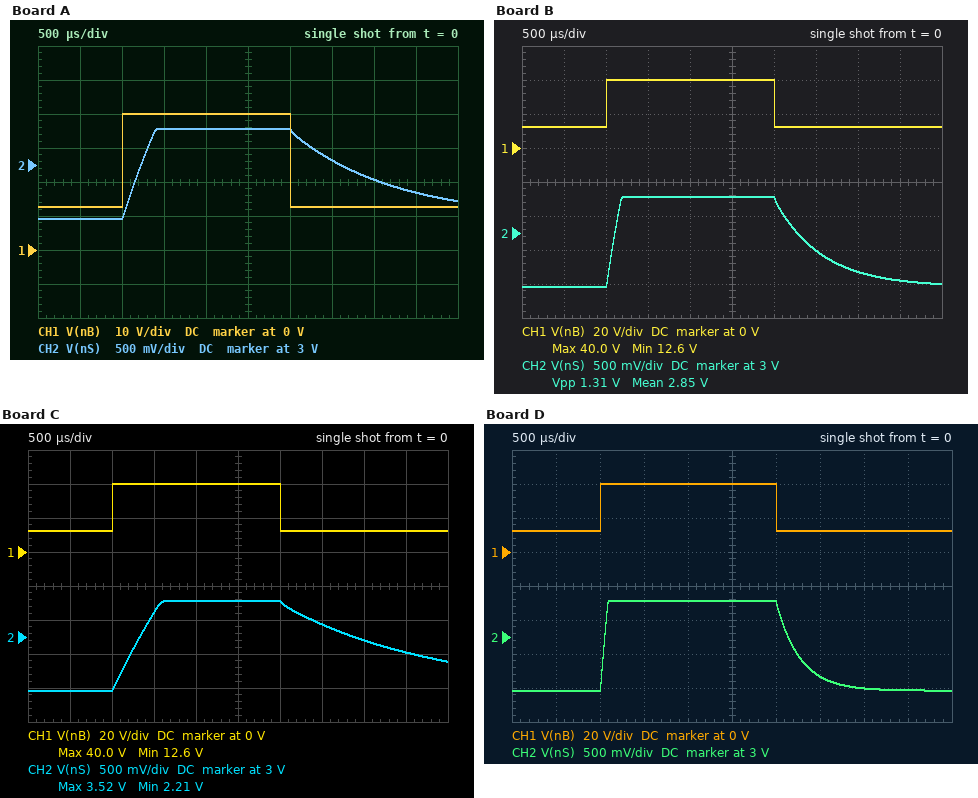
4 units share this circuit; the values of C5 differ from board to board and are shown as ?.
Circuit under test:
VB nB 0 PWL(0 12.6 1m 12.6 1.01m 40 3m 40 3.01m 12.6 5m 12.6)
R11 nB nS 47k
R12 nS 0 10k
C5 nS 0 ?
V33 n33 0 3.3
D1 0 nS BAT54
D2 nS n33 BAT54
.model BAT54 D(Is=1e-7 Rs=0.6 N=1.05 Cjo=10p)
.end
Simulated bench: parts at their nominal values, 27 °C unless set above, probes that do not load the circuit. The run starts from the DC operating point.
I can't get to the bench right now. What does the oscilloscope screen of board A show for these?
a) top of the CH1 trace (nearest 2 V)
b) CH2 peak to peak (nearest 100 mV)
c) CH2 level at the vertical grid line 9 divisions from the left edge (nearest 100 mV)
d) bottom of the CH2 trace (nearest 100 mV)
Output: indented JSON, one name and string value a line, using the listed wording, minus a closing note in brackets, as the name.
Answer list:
{
  "top of the CH1 trace": "40 V",
  "CH2 peak to peak": "1.3 V",
  "CH2 level at the vertical grid line 9 divisions from the left edge": "2.6 V",
  "bottom of the CH2 trace": "2.2 V"
}
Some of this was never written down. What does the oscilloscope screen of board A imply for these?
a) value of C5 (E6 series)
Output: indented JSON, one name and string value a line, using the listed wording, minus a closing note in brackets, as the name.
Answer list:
{
  "value of C5": "150 nF"
}
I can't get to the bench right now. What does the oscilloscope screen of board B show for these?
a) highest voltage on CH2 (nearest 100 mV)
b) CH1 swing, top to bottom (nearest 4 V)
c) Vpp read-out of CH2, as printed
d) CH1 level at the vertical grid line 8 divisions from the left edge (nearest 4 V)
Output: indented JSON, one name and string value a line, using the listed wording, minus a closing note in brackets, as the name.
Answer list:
{
  "highest voltage on CH2": "3.5 V",
  "CH1 swing, top to bottom": "28 V",
  "Vpp read-out of CH2, as printed": "1.31 V",
  "CH1 level at the vertical grid line 8 divisions from the left edge": "12 V"
}
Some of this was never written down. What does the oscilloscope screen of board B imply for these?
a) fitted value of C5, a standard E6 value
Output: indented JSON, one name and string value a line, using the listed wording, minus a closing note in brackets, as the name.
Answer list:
{
  "fitted value of C5, a standard E6 value": "68 nF"
}
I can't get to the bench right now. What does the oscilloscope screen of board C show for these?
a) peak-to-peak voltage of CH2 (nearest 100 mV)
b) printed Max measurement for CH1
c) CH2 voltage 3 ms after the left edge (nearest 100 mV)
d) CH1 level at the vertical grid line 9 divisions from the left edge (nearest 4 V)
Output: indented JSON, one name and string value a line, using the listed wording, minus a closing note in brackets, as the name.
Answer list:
{
  "peak-to-peak voltage of CH2": "1.3 V",
  "printed Max measurement for CH1": "40.0 V",
  "CH2 voltage 3 ms after the left edge": "3.5 V",
  "CH1 level at the vertical grid line 9 divisions from the left edge": "12 V"
}
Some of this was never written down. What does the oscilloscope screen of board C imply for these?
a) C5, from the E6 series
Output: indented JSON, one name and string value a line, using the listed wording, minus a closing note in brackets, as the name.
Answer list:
{
  "C5, from the E6 series": "220 nF"
}
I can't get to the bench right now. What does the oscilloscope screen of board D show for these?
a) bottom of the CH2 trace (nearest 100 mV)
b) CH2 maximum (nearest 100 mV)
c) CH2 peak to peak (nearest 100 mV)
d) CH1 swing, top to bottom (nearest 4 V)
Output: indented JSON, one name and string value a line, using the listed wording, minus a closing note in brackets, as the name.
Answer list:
{
  "bottom of the CH2 trace": "2.2 V",
  "CH2 maximum": "3.5 V",
  "CH2 peak to peak": "1.3 V",
  "CH1 swing, top to bottom": "28 V"
}
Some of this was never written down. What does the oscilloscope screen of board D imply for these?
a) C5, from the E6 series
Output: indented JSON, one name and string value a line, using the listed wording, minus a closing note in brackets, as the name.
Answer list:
{
  "C5, from the E6 series": "33 nF"
}
